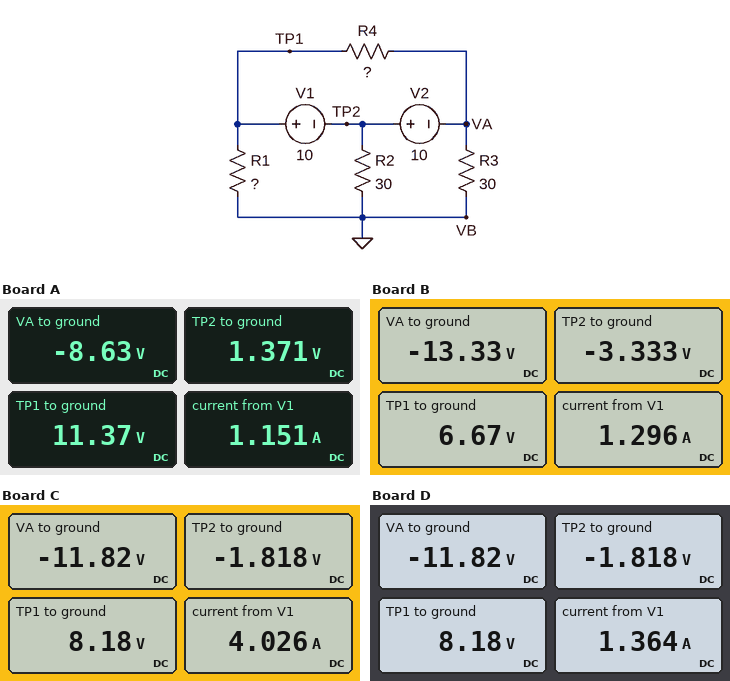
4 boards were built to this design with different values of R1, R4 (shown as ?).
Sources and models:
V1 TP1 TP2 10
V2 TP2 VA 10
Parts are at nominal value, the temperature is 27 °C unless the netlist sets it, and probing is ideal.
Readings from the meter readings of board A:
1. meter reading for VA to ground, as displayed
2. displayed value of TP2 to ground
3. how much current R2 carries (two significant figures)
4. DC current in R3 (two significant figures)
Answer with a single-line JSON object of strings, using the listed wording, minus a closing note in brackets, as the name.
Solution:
{"meter reading for VA to ground, as displayed": "-8.63 V", "displayed value of TP2 to ground": "1.371 V", "how much current R2 carries": "46 mA", "DC current in R3": "290 mA"}
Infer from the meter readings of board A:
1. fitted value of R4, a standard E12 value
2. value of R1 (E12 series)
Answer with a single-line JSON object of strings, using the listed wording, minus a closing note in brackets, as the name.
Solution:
{"fitted value of R4, a standard E12 value": "22 Ω", "value of R1": "47 Ω"}
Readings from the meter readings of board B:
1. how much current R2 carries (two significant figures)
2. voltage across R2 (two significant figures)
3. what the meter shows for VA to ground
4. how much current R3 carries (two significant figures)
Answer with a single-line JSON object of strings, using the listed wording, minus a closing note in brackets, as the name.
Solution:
{"how much current R2 carries": "110 mA", "voltage across R2": "3.3 V", "what the meter shows for VA to ground": "-13.33 V", "how much current R3 carries": "440 mA"}
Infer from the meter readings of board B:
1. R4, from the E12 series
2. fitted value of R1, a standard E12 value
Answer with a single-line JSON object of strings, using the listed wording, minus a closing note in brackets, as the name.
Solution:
{"R4, from the E12 series": "27 Ω", "fitted value of R1, a standard E12 value": "12 Ω"}
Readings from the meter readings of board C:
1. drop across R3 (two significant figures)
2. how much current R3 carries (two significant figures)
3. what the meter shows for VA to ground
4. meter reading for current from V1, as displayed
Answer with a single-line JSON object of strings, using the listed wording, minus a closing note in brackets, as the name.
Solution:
{"drop across R3": "12 V", "how much current R3 carries": "390 mA", "what the meter shows for VA to ground": "-11.82 V", "meter reading for current from V1, as displayed": "4.026 A"}
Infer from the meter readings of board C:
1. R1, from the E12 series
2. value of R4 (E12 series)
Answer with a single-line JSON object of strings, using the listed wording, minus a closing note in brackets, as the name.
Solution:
{"R1, from the E12 series": "18 Ω", "value of R4": "5.6 Ω"}
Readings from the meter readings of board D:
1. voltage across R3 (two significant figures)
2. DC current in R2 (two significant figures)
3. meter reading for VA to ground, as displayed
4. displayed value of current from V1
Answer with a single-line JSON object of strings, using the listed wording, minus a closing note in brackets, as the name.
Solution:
{"voltage across R3": "12 V", "DC current in R2": "61 mA", "meter reading for VA to ground, as displayed": "-11.82 V", "displayed value of current from V1": "1.364 A"}
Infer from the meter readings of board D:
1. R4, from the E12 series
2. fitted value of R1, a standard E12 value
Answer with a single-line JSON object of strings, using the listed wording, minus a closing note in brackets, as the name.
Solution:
{"R4, from the E12 series": "22 Ω", "fitted value of R1, a standard E12 value": "18 Ω"}
